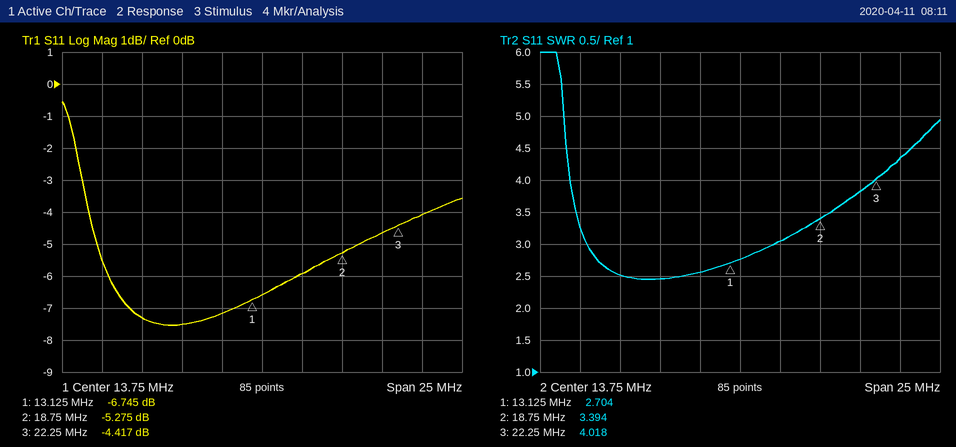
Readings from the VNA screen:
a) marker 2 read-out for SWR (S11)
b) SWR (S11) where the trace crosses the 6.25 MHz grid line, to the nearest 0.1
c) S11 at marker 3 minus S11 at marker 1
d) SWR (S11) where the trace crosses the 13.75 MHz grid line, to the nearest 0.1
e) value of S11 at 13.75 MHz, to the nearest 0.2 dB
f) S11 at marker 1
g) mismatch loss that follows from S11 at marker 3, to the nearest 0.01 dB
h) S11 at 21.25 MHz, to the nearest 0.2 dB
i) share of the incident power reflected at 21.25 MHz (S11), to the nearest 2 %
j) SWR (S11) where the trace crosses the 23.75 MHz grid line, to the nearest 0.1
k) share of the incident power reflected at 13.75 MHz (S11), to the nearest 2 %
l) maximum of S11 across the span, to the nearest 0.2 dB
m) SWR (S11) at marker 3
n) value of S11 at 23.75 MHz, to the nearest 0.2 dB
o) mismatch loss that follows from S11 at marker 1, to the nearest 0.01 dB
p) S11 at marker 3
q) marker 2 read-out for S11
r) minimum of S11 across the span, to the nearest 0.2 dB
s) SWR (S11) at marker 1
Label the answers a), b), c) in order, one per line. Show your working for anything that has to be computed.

a) 3.394
b) 2.5
c) -4.417 − (-6.745) = 2.328 dB
d) 2.8
e) -6.6 dB
f) -6.745 dB
g) −10 log10(1 − 10^(-4.417/10)) ≈ 1.95 dB
h) -4.6 dB
i) 10^(-4.6/10) ≈ 34.7 %, so 34 % to the nearest 2 %
j) 4.3
k) 10^(-6.6/10) ≈ 22 %
l) -0.6 dB
m) 4.018
n) -4.0 dB
o) −10 log10(1 − 10^(-6.745/10)) ≈ 1.03 dB
p) -4.417 dB
q) -5.275 dB
r) -7.6 dB
s) 2.704
